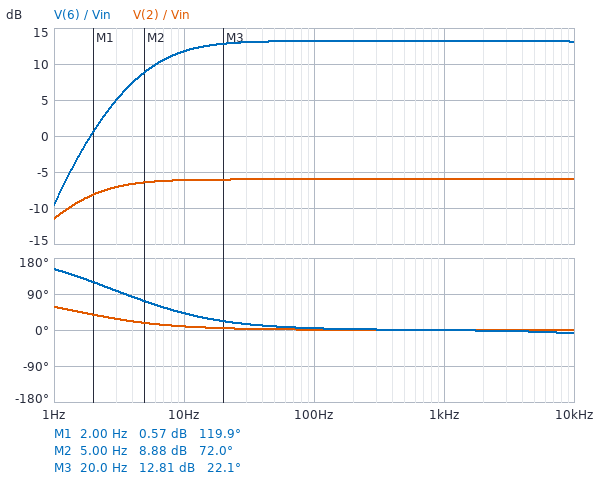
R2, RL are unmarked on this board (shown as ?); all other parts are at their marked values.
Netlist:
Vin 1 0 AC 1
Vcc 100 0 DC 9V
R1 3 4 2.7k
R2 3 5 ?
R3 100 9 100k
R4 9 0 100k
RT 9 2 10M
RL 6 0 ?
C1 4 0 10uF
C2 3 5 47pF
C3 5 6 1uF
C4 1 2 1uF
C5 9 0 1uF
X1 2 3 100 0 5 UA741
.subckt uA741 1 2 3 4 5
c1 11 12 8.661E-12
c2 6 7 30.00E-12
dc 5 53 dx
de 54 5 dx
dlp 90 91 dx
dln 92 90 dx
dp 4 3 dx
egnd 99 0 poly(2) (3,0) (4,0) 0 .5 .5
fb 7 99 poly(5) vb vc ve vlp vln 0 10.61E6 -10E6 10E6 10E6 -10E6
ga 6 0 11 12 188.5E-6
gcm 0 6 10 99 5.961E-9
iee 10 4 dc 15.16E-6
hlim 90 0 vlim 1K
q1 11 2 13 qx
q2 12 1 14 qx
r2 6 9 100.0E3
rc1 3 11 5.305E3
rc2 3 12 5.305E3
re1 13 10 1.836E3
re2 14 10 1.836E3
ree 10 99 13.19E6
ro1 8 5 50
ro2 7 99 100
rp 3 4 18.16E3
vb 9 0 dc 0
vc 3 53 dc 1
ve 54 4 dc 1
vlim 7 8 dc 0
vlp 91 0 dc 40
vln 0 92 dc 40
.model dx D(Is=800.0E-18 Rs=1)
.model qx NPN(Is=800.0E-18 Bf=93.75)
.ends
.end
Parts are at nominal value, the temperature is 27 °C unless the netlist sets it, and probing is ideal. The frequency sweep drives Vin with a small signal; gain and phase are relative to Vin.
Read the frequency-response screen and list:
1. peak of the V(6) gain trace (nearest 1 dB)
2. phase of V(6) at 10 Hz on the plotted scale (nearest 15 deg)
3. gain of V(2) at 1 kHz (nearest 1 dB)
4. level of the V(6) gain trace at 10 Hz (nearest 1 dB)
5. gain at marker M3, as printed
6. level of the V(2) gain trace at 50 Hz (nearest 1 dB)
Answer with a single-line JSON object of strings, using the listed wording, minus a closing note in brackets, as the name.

{"peak of the V(6) gain trace": "13 dB", "phase of V(6) at 10 Hz on the plotted scale": "45 deg", "gain of V(2) at 1 kHz": "-6 dB", "level of the V(6) gain trace at 10 Hz": "12 dB", "gain at marker M3, as printed": "12.81 dB", "level of the V(2) gain trace at 50 Hz": "-6 dB"}
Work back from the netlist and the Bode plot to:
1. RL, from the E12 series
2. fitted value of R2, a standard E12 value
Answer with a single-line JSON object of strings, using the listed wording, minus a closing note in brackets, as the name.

{"RL, from the E12 series": "150 kΩ", "fitted value of R2, a standard E12 value": "22 kΩ"}
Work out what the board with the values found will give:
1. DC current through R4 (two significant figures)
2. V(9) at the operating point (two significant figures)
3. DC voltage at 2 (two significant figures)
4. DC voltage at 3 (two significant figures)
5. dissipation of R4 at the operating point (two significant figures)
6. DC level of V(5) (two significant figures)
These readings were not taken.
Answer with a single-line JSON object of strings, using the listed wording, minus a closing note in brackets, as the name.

{"DC current through R4": "45 µA", "V(9) at the operating point": "4.5 V", "DC voltage at 2": "4.5 V", "DC voltage at 3": "4.5 V", "dissipation of R4 at the operating point": "200 µW", "DC level of V(5)": "4.5 V"}
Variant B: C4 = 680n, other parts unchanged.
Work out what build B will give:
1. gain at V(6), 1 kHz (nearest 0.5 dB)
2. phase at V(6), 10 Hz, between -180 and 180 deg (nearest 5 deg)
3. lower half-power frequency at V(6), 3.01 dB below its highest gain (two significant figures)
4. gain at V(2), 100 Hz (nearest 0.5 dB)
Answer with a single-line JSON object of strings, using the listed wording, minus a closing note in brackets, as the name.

{"gain at V(6), 1 kHz": "11.5 dB", "phase at V(6), 10 Hz, between -180 and 180 deg": "45 deg", "lower half-power frequency at V(6), 3.01 dB below its highest gain": "6.5 Hz", "gain at V(2), 100 Hz": "-8.0 dB"}
